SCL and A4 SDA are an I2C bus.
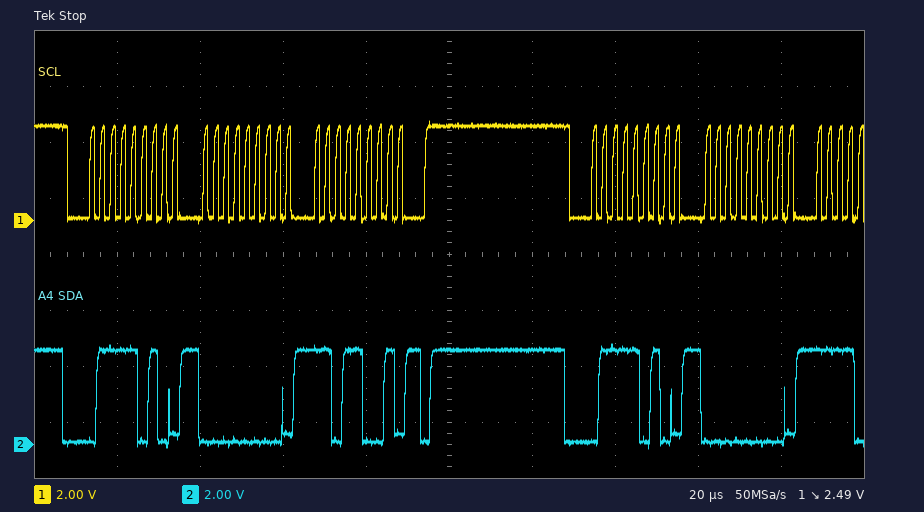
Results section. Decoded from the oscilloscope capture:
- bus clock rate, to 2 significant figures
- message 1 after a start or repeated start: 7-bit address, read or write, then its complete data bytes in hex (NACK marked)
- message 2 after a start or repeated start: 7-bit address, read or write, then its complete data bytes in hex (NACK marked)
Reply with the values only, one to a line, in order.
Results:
400 kHz
0x3D write: 00 D9
0x3D write: 00
